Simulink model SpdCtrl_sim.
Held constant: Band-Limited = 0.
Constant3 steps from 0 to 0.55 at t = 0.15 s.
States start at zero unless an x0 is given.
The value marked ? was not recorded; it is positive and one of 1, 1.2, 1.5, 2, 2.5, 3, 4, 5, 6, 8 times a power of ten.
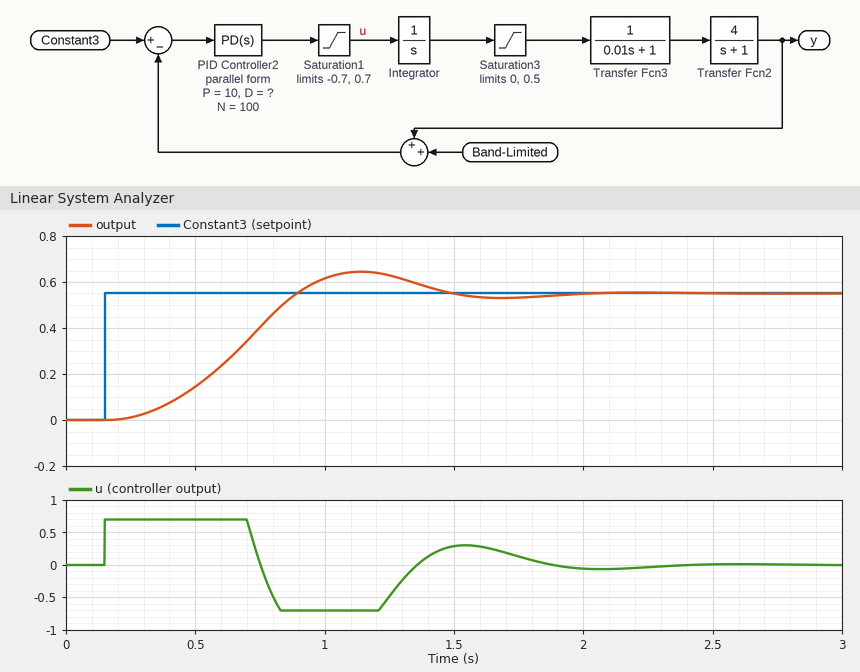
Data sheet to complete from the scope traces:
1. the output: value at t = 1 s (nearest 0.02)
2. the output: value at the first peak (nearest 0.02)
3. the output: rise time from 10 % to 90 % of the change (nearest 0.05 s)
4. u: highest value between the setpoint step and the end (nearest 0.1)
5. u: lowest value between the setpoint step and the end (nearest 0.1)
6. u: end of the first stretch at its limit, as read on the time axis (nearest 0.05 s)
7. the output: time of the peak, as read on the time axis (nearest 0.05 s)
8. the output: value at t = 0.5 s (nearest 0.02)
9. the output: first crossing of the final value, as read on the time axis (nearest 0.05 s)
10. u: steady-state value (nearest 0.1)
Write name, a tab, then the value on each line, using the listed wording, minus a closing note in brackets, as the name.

the output: value at t = 1 s	0.62
the output: value at the first peak	0.64
the output: rise time from 10 % to 90 % of the change	0.45 s
u: highest value between the setpoint step and the end	0.7
u: lowest value between the setpoint step and the end	-0.7
u: end of the first stretch at its limit, as read on the time axis	0.70 s
the output: time of the peak, as read on the time axis	1.15 s
the output: value at t = 0.5 s	0.14
the output: first crossing of the final value, as read on the time axis	0.90 s
u: steady-state value	0.0
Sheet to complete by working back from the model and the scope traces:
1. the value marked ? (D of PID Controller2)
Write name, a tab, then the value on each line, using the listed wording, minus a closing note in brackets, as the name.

the value marked ?	1.2
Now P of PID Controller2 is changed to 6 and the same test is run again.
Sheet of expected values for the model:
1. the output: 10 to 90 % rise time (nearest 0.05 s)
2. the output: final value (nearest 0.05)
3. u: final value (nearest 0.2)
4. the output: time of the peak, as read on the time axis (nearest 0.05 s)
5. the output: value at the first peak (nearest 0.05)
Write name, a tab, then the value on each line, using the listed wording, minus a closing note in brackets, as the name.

the output: 10 to 90 % rise time	0.50 s
the output: final value	0.55
u: final value	0.0
the output: time of the peak, as read on the time axis	1.20 s
the output: value at the first peak	0.60
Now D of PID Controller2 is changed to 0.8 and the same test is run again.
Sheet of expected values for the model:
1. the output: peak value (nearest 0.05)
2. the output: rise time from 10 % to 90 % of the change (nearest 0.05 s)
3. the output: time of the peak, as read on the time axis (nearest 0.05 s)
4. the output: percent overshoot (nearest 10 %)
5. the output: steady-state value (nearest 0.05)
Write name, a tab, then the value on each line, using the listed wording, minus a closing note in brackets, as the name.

the output: peak value	0.70
the output: rise time from 10 % to 90 % of the change	0.45 s
the output: time of the peak, as read on the time axis	1.20 s
the output: percent overshoot	30 %
the output: steady-state value	0.55
